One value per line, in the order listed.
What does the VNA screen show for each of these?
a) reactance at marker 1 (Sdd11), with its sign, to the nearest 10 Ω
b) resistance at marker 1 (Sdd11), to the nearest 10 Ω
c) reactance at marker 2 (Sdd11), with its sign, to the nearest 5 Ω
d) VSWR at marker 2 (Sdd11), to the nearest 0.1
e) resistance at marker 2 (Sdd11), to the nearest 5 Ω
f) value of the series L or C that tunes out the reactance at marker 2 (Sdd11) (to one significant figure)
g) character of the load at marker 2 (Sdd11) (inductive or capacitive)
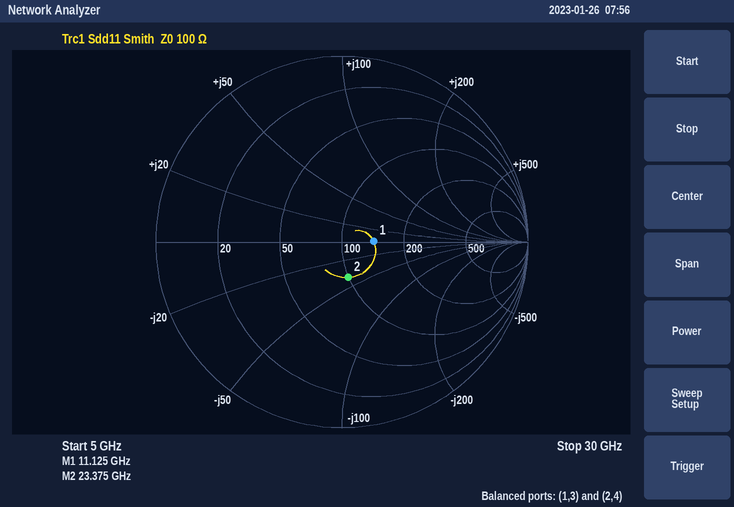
0 Ω
140 Ω
-40 Ω
1.5
100 Ω
300 pH
capacitive
